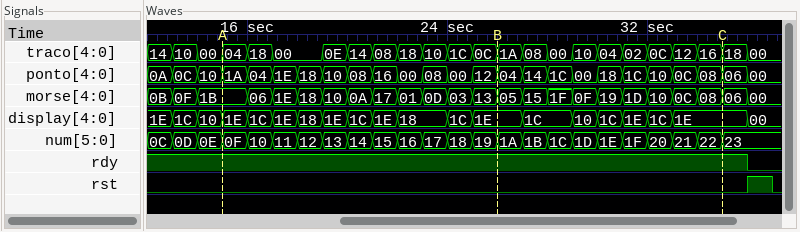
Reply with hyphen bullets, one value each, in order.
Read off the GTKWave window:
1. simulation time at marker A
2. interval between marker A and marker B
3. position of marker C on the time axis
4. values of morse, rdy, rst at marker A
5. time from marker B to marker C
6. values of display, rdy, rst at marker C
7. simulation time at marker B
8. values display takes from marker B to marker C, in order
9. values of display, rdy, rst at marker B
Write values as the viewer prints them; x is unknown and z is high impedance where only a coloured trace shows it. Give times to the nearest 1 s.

- 15 s
- 11 s
- 35 s
- morse=1B, rdy=1, rst=0
- 9 s
- display=1E, rdy=1, rst=0
- 26 s
- 1E, 1C, 10, 1C, 1E, 1C, 1E
- display=1E, rdy=1, rst=0
